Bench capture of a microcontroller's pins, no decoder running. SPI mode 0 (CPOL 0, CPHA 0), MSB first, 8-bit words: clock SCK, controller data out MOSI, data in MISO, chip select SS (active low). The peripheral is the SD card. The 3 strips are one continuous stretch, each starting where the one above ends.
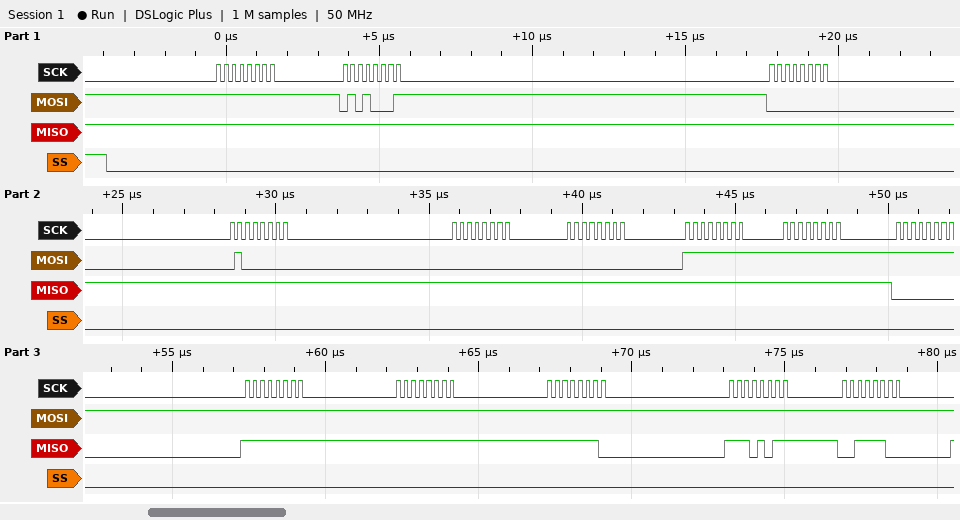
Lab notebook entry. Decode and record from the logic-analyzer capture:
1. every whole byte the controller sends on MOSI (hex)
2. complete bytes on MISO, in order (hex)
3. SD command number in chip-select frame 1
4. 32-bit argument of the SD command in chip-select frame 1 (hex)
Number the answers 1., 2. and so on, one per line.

1. FF 51 00 40 00 00 FF FF FF FF FF FF FF FF
2. FF FF FF FF FF FF FF FF 00 FF FF FE EB 3C
3. CMD17
4. 0x00400000
